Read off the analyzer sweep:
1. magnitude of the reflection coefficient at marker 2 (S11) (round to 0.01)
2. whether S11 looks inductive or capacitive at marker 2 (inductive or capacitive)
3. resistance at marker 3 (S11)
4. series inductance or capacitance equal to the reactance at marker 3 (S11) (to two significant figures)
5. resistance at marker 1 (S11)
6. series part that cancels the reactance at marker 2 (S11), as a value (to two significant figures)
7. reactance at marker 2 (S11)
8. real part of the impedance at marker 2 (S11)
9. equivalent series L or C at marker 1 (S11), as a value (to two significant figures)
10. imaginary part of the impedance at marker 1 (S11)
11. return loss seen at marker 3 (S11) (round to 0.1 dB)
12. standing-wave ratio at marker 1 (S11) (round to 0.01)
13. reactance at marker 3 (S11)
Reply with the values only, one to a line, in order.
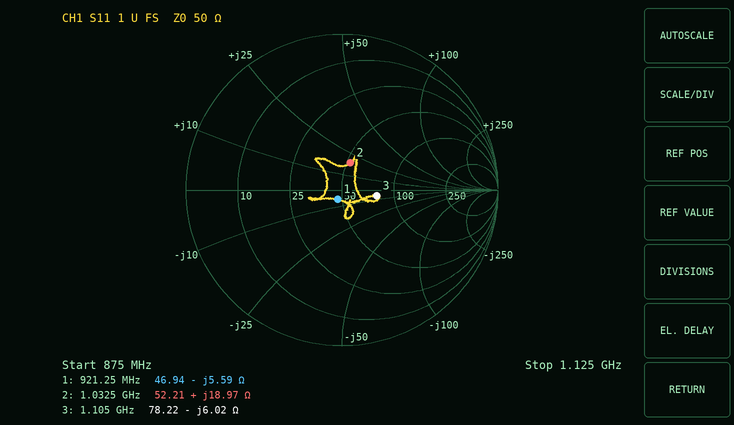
0.18
inductive
78.22 Ω
24 pF
46.94 Ω
8.1 pF
+18.97 Ω
52.21 Ω
31 pF
-5.59 Ω
13.0 dB
1.14
-6.02 Ω
